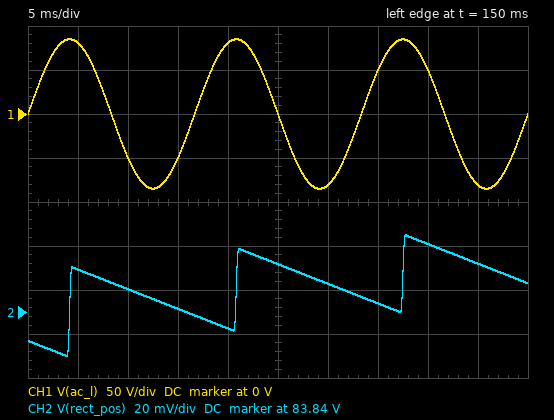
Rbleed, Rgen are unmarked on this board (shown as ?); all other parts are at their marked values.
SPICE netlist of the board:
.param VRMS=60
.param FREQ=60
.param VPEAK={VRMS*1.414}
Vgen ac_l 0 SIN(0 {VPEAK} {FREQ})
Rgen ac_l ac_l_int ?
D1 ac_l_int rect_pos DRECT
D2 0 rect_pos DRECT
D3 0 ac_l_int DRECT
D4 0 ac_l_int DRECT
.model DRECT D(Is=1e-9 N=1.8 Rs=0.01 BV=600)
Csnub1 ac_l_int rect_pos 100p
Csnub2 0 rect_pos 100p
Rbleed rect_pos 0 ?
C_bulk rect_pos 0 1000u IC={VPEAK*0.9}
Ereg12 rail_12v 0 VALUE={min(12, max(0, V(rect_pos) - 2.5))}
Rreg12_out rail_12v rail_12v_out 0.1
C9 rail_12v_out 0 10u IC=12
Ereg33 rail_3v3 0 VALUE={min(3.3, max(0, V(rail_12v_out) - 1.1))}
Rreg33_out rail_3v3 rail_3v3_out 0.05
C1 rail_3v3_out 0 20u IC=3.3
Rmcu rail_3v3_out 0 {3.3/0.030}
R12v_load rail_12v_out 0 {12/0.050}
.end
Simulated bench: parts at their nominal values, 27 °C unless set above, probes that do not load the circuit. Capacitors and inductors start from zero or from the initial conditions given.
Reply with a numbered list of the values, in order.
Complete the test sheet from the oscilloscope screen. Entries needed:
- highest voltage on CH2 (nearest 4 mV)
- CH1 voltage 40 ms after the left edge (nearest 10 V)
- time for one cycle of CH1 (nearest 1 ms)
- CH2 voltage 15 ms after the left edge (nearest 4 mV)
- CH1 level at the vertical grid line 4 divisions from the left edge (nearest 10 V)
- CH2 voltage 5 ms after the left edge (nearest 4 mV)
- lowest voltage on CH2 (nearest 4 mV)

1. 83.876 V
2. 50 V
3. 17 ms
4. 83.840 V
5. 80 V
6. 83.860 V
7. 83.820 V
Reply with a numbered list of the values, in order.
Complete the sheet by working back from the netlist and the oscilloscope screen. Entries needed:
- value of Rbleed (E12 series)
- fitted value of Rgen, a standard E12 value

1. 47 kΩ
2. 0.68 Ω
